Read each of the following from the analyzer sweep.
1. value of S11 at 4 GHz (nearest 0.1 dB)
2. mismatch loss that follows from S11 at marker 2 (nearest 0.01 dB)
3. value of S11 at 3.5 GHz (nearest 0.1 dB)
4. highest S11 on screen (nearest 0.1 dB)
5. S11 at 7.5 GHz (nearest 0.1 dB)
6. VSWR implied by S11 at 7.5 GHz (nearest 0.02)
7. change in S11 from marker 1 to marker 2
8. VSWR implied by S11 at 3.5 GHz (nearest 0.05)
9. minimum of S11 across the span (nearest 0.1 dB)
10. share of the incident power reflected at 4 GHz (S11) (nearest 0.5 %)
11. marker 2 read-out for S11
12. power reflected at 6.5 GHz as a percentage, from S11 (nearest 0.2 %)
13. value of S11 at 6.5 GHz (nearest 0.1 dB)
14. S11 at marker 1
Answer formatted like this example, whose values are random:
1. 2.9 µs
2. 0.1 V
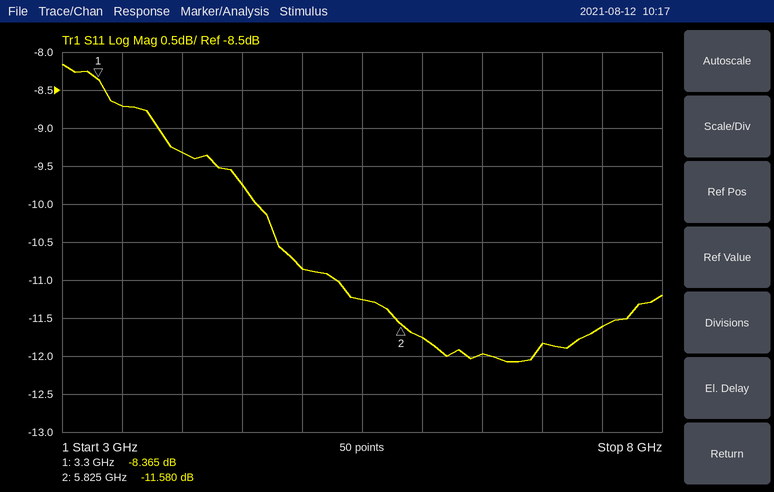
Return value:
1. -9.3 dB
2. 0.31 dB
3. -8.7 dB
4. -8.2 dB
5. -11.6 dB
6. 1.72
7. -3.215 dB
8. 2.15
9. -12.1 dB
10. 11.5 %
11. -11.580 dB
12. 6.4 %
13. -12.0 dB
14. -8.365 dB
